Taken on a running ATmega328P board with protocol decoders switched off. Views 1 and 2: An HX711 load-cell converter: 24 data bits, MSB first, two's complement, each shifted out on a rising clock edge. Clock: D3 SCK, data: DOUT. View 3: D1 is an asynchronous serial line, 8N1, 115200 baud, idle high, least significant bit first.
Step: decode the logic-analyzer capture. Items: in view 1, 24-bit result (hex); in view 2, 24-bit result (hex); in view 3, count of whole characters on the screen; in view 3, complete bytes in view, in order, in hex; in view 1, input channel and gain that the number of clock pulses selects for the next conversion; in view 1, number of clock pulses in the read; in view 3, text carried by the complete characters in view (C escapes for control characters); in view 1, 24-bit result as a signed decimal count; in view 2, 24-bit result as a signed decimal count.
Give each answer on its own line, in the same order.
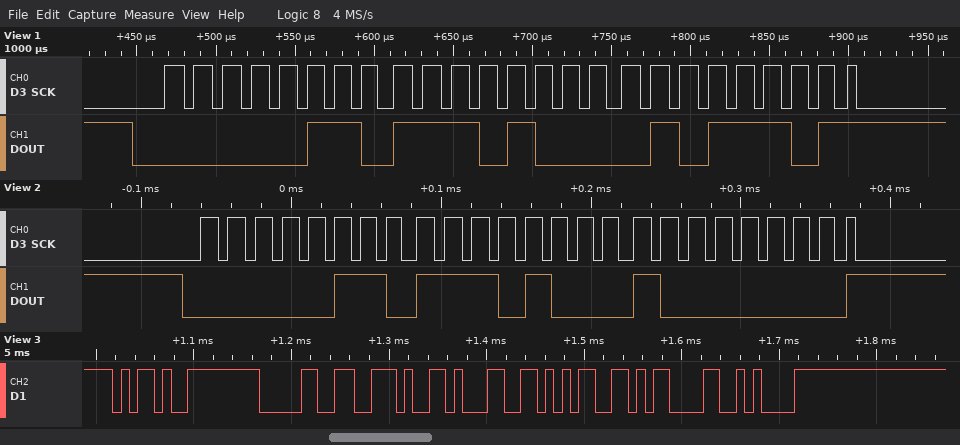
0x06E85D
0x06E880
7
0x2D 0x30 0x2E 0x31 0x35 0x0D 0x0A
channel A, gain 128
25
"-0.15\r\n"
452701
452736
